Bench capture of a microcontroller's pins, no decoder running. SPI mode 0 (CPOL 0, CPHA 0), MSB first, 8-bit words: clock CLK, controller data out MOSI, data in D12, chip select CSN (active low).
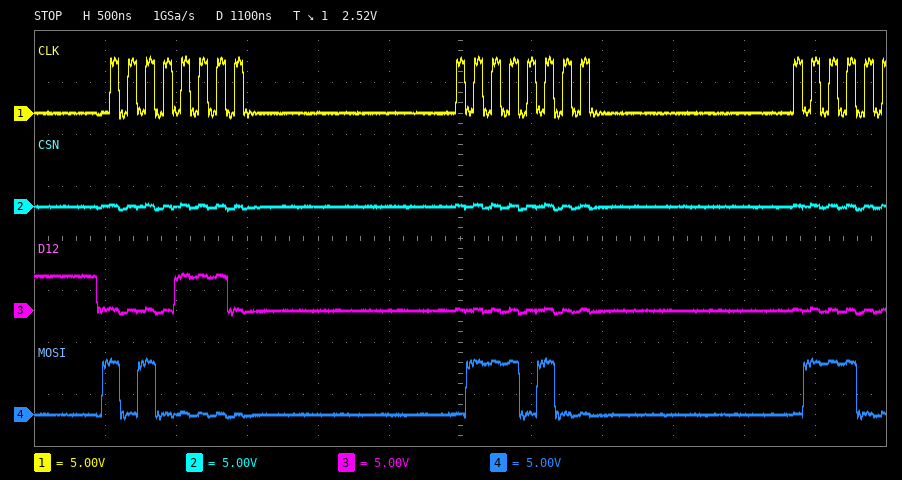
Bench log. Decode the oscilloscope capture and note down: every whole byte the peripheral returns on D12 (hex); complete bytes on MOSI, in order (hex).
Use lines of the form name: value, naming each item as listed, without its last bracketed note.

every whole byte the peripheral returns on D12: 0E 00
complete bytes on MOSI, in order: A0 74
